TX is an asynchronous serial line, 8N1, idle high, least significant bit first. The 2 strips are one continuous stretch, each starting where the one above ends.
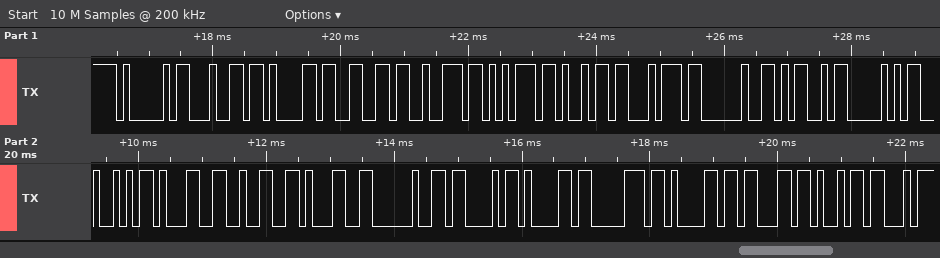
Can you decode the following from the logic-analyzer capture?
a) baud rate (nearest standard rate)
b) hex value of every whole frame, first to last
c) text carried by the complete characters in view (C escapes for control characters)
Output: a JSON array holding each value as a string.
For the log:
["9600 baud", "41 64 61 66 72 75 69 74 20 4D 50 52 31 32 31 20 43 61 70 61 63 69", "\"Adafruit MPR121 Capaci\""]
